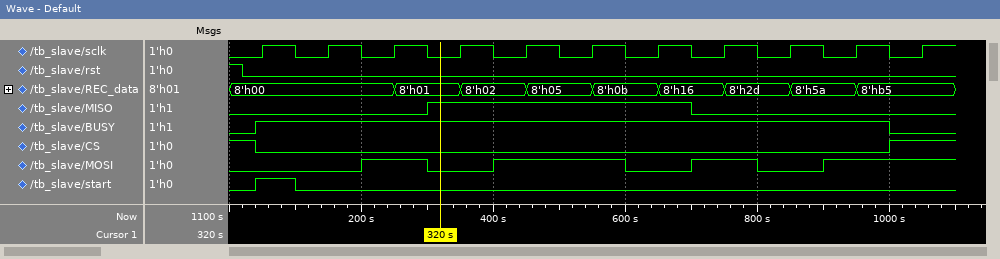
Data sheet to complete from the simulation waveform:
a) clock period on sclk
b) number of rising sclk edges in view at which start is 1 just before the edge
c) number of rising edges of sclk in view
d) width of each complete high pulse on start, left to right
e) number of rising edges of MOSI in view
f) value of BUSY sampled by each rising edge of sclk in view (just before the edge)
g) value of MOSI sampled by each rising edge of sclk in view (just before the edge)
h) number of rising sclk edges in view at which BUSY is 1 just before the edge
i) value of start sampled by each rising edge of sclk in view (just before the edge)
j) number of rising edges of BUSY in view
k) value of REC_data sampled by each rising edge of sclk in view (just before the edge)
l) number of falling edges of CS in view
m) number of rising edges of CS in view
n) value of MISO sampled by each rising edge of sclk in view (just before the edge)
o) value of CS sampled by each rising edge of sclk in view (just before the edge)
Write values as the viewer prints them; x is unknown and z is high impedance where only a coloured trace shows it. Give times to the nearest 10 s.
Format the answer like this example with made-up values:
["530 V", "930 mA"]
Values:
["100 s", "1", "11", "60 s", "4", "1 1 1 1 1 1 1 1 1 1 0", "0 0 1 0 1 1 0 1 0 1 1", "10", "1 0 0 0 0 0 0 0 0 0 0", "1", "8'h00, 8'h00, 8'h00, 8'h01, 8'h02, 8'h05, 8'h0b, 8'h16, 8'h2d, 8'h5a, 8'hb5", "1", "1", "0 0 0 1 1 1 1 0 0 0 0", "0 0 0 0 0 0 0 0 0 0 1"]
